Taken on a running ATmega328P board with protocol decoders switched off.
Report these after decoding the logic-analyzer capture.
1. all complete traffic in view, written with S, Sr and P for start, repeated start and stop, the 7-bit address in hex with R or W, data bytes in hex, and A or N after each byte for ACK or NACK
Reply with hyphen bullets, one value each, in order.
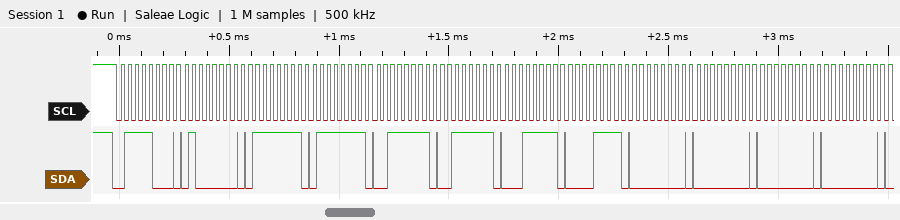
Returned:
- S 3CW A 40 A 7F A 7F A 3F A 3F A 1F A 0F A 00 A 00 A 00 A 00 A
